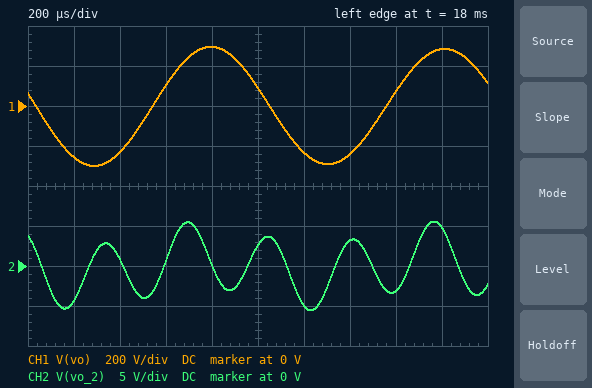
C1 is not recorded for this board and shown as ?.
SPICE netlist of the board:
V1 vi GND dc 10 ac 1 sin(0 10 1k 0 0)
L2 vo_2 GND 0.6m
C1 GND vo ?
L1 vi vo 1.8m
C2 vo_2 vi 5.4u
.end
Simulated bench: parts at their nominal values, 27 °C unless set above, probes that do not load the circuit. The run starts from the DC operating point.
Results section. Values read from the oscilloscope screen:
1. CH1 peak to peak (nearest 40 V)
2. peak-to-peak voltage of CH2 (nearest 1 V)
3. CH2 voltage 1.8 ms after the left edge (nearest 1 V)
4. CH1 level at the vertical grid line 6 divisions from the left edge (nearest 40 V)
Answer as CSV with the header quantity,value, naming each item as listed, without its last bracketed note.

quantity,value
CH1 peak to peak,600 V
peak-to-peak voltage of CH2,11 V
CH2 voltage 1.8 ms after the left edge,5 V
CH1 level at the vertical grid line 6 divisions from the left edge,-240 V
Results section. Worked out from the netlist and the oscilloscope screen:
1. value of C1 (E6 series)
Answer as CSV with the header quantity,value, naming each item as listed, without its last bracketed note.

quantity,value
value of C1,15 µF
